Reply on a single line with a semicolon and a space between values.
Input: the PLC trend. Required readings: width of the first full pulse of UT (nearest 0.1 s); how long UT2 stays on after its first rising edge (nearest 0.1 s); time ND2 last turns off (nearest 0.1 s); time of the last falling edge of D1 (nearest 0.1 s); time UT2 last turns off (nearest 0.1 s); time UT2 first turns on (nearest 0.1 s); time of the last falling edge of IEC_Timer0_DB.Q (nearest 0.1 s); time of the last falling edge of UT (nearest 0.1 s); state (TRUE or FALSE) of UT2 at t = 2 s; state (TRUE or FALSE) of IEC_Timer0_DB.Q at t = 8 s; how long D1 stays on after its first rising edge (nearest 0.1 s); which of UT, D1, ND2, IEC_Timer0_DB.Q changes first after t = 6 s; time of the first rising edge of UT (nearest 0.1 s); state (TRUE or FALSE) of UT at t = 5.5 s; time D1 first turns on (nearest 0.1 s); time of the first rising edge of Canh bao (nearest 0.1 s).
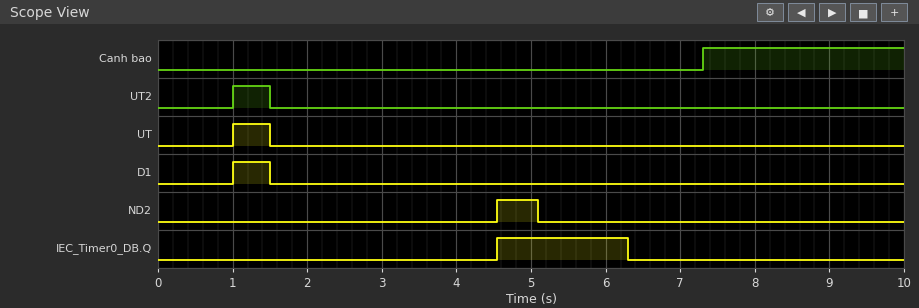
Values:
0.5 s; 0.5 s; 5.1 s; 1.5 s; 1.5 s; 1.0 s; 6.3 s; 1.5 s; FALSE; FALSE; 0.5 s; IEC_Timer0_DB.Q; 1.0 s; FALSE; 1.0 s; 7.3 s
